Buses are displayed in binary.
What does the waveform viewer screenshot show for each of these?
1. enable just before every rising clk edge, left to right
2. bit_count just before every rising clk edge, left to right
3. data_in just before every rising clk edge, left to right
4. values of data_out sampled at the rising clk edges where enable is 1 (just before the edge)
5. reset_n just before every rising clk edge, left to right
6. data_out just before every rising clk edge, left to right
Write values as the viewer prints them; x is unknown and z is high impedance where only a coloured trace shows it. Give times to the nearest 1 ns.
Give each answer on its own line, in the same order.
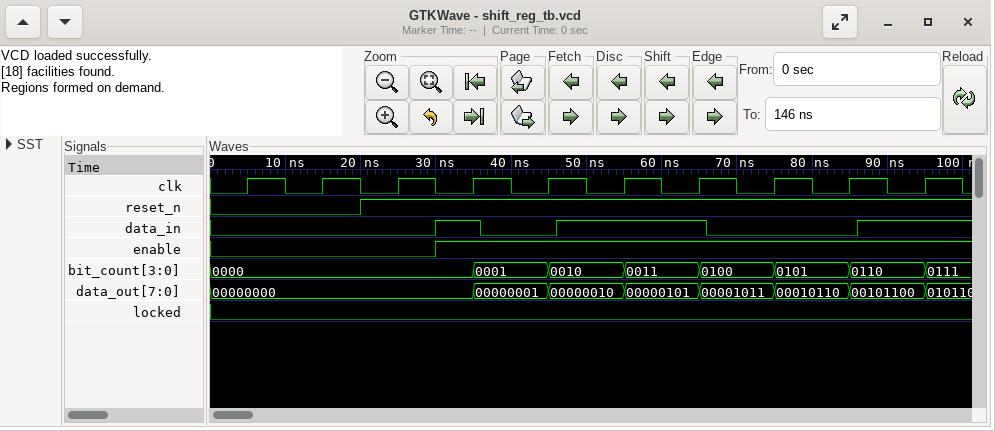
0 0 0 1 1 1 1 1 1 1
0000, 0000, 0000, 0000, 0001, 0010, 0011, 0100, 0101, 0110
0 0 0 1 0 1 1 0 0 1
00000000, 00000001, 00000010, 00000101, 00001011, 00010110, 00101100
0 0 1 1 1 1 1 1 1 1
00000000, 00000000, 00000000, 00000000, 00000001, 00000010, 00000101, 00001011, 00010110, 00101100
